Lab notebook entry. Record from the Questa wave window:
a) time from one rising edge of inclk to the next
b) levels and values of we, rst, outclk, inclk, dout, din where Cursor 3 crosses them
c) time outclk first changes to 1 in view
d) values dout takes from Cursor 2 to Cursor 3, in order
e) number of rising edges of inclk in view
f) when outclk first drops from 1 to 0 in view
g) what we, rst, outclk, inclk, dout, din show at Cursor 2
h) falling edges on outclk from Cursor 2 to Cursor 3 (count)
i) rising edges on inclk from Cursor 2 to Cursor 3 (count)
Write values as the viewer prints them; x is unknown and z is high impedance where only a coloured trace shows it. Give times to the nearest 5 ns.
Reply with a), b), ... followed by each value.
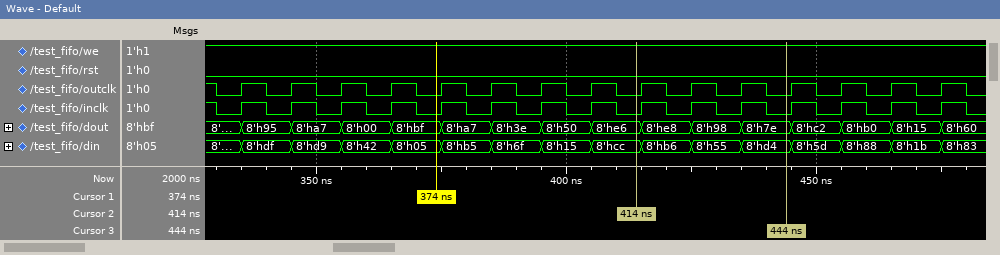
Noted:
a) 10 ns
b) we=1, rst=0, outclk=0, inclk=0, dout=8'h7e, din=8'hd4
c) 335 ns
d) 8'he6, 8'he8, 8'h98, 8'h7e
e) 15
f) 330 ns
g) we=1, rst=0, outclk=0, inclk=0, dout=8'he6, din=8'hcc
h) 3
i) 3
